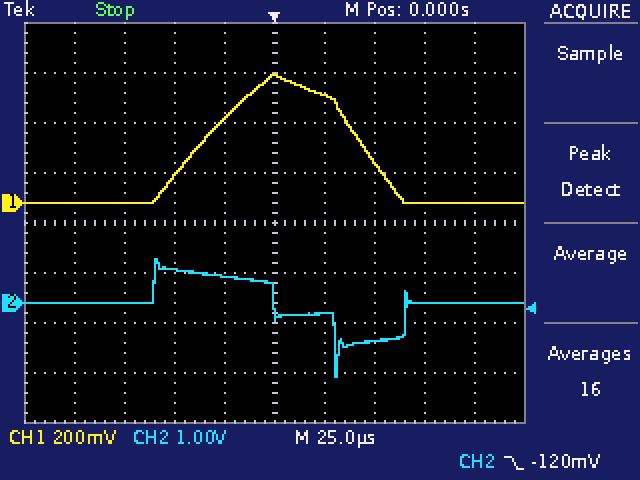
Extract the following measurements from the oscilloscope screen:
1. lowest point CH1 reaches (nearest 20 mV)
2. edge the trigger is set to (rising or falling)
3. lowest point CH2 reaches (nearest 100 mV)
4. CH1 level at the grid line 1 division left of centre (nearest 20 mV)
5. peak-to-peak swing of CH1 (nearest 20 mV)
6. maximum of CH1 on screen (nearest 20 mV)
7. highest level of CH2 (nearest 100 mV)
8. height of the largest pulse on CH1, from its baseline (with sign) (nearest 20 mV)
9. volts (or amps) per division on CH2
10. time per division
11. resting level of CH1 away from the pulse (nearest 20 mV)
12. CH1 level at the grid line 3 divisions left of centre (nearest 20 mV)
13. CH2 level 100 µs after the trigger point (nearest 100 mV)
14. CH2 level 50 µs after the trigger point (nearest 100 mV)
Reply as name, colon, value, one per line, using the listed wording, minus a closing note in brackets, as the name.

lowest point CH1 reaches: 0 mV
edge the trigger is set to: falling
lowest point CH2 reaches: -1.5 V
CH1 level at the grid line 1 division left of centre: 340 mV
peak-to-peak swing of CH1: 520 mV
maximum of CH1 on screen: 520 mV
highest level of CH2: 900 mV
height of the largest pulse on CH1, from its baseline (with sign): +520 mV
volts (or amps) per division on CH2: 1 V
time per division: 25 µs
resting level of CH1 away from the pulse: 0 mV
CH1 level at the grid line 3 divisions left of centre: 0 mV
CH2 level 100 µs after the trigger point: 0.0 V
CH2 level 50 µs after the trigger point: -800 mV
